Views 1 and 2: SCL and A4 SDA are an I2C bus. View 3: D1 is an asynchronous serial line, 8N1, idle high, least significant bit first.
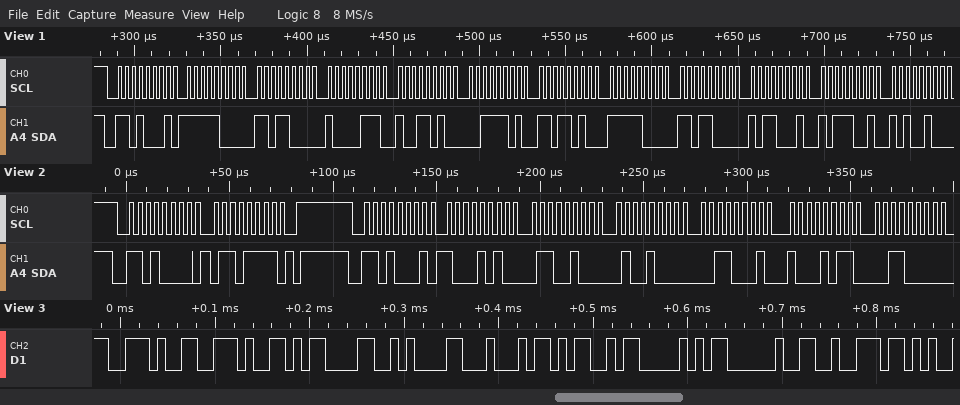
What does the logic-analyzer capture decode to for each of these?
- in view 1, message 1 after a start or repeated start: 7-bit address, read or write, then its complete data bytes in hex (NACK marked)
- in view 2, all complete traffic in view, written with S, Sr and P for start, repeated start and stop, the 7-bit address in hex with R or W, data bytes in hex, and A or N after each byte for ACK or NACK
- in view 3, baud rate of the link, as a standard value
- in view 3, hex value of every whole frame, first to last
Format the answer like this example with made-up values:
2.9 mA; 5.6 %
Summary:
0x68 read: F8 D8 87 9A 3D DA F8 D8 B1 B9 A4; S 68W A 6F A P S 68R A 8A A 64 A 48 A 31 A 8B A 30 A; 115200 baud; 0x2E 0x2E 0x0D 0x0A 0x44 0x4D 0x50 0x20 0x72
